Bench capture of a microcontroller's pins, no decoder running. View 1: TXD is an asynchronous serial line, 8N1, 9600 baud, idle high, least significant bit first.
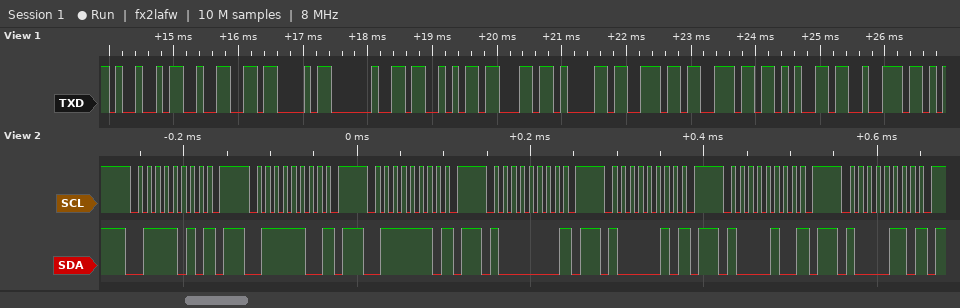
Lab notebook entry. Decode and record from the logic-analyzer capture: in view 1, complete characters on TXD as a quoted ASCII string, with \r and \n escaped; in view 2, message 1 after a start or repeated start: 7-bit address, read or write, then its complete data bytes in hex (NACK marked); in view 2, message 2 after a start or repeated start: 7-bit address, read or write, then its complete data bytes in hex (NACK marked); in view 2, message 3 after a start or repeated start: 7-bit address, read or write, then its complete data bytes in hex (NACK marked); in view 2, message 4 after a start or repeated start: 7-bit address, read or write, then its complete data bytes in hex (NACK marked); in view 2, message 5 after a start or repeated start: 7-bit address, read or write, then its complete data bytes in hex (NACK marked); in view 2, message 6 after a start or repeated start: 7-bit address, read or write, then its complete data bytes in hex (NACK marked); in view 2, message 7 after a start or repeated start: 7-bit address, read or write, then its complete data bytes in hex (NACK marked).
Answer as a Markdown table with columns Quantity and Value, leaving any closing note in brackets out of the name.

| Quantity | Value |
|---|---|
| in view 1, complete characters on TXD as a quoted ASCII string, with \r and \n escaped | "I2C Scanner" |
| in view 2, message 1 after a start or repeated start: 7-bit address, read or write, then its complete data bytes in hex | 0x3D write NACK |
| in view 2, message 2 after a start or repeated start: 7-bit address, read or write, then its complete data bytes in hex | 0x3E write NACK |
| in view 2, message 3 after a start or repeated start: 7-bit address, read or write, then its complete data bytes in hex | 0x3F write NACK |
| in view 2, message 4 after a start or repeated start: 7-bit address, read or write, then its complete data bytes in hex | 0x40 write NACK |
| in view 2, message 5 after a start or repeated start: 7-bit address, read or write, then its complete data bytes in hex | 0x41 write NACK |
| in view 2, message 6 after a start or repeated start: 7-bit address, read or write, then its complete data bytes in hex | 0x42 write NACK |
| in view 2, message 7 after a start or repeated start: 7-bit address, read or write, then its complete data bytes in hex | 0x43 write NACK |
